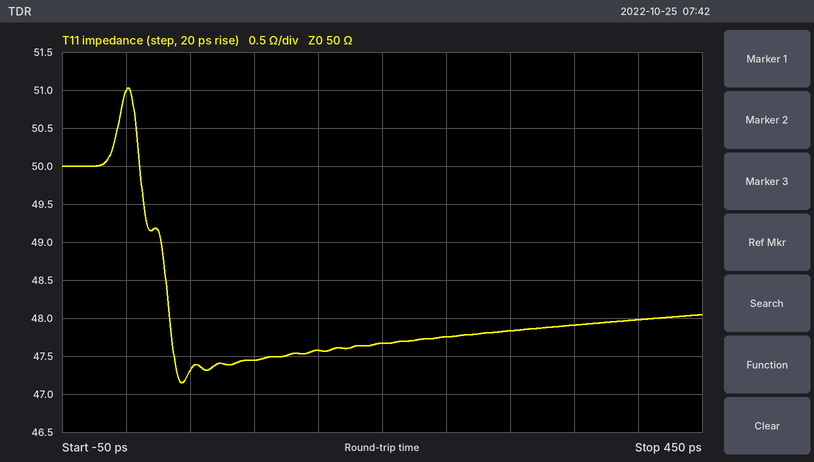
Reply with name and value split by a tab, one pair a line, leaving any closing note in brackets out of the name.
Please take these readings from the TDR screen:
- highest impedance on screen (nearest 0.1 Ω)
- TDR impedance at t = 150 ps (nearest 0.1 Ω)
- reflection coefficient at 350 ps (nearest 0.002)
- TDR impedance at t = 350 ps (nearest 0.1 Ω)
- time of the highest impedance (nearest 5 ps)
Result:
highest impedance on screen	51.0 Ω
TDR impedance at t = 150 ps	47.6 Ω
reflection coefficient at 350 ps	-0.022
TDR impedance at t = 350 ps	47.9 Ω
time of the highest impedance	0 ps
